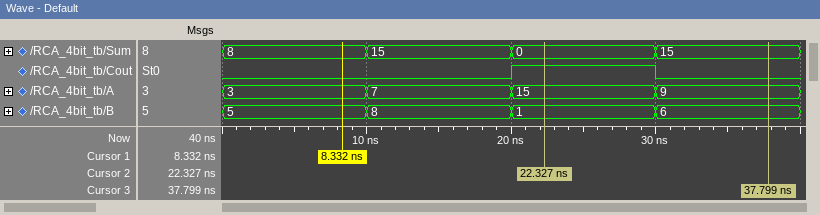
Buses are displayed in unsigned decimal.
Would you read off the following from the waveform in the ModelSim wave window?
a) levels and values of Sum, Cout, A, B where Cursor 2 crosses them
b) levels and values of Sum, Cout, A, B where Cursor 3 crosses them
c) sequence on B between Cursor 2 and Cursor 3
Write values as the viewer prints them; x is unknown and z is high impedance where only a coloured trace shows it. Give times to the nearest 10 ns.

Sum=0, Cout=1, A=15, B=1
Sum=15, Cout=0, A=9, B=6
1, 6
